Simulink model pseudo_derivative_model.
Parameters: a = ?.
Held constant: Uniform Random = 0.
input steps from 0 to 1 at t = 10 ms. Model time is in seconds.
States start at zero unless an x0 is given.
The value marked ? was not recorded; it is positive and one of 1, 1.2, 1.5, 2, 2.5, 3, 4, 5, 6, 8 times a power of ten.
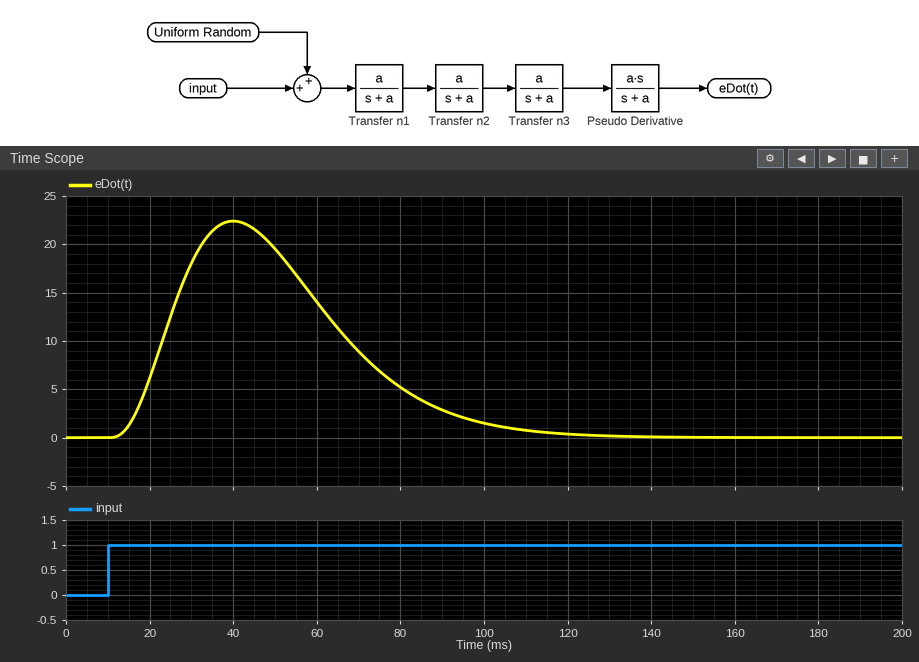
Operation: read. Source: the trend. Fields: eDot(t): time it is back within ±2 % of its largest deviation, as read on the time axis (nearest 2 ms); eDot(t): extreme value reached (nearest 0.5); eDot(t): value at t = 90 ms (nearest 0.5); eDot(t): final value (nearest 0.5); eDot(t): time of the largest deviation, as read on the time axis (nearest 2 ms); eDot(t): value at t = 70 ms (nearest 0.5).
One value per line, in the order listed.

118 ms
22.5
3.0
0.0
40 ms
9.0
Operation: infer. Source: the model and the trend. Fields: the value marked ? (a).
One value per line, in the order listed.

100
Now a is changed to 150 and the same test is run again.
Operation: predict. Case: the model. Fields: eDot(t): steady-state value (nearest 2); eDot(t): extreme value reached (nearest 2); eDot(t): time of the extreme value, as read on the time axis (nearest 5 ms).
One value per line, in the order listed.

0
34
30 ms
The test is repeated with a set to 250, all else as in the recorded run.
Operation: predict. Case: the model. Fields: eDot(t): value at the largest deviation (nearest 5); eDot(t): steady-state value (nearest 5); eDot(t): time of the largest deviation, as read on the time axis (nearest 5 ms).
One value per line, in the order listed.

55
0
20 ms
